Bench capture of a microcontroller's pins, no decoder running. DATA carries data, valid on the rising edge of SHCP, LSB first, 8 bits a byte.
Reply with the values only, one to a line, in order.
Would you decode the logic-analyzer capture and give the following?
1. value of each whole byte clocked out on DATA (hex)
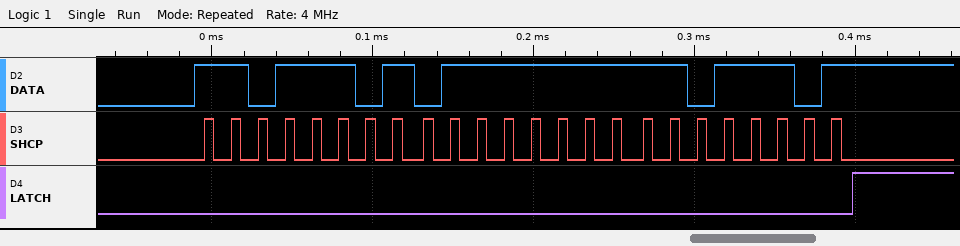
BB FE BB
